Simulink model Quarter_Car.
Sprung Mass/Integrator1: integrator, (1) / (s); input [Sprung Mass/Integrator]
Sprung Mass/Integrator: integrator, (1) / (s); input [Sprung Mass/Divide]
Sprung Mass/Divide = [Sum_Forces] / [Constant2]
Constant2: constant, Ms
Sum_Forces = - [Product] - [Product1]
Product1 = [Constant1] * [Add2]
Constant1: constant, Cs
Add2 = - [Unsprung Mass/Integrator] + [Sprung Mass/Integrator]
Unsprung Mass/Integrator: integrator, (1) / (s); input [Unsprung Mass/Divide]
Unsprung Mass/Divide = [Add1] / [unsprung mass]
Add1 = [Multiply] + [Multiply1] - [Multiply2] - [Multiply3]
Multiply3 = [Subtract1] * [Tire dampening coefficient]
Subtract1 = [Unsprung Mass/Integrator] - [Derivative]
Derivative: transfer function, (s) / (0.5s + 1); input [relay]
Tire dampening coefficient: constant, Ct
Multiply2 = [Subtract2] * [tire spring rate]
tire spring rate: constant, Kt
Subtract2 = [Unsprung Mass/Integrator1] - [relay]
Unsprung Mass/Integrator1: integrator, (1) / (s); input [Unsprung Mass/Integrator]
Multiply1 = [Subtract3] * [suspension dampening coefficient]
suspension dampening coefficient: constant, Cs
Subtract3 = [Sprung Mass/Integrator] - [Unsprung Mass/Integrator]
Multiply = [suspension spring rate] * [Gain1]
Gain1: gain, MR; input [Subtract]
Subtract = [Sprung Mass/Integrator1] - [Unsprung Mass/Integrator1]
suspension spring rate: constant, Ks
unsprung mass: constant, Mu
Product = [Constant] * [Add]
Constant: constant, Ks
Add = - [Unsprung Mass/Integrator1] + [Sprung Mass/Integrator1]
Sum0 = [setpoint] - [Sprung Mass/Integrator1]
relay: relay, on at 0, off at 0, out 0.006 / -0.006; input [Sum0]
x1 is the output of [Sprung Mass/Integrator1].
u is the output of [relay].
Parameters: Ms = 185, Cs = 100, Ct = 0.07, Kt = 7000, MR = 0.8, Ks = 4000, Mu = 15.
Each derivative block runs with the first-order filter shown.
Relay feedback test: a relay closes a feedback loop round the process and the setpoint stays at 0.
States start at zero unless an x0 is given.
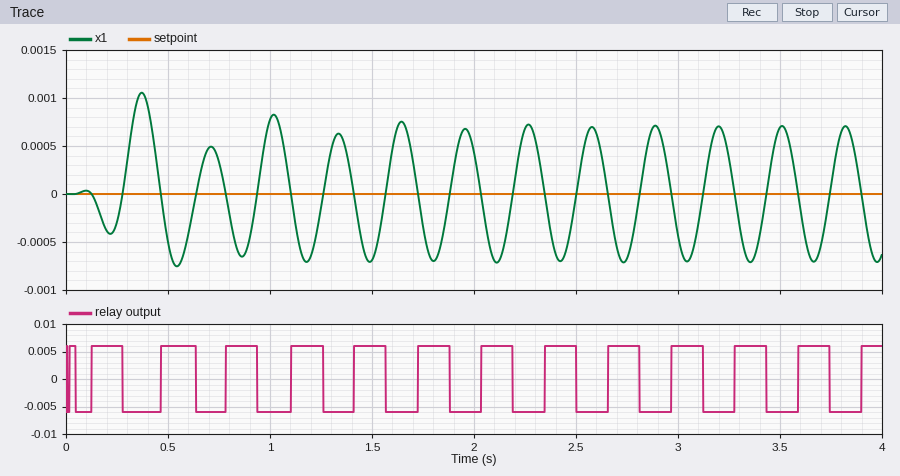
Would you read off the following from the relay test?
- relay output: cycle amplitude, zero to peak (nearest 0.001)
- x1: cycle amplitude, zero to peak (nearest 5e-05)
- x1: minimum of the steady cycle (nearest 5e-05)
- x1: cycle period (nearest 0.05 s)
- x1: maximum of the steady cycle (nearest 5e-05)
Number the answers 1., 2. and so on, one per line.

1. 0.006
2. 0.00070
3. -0.00070
4. 0.30 s
5. 0.00070
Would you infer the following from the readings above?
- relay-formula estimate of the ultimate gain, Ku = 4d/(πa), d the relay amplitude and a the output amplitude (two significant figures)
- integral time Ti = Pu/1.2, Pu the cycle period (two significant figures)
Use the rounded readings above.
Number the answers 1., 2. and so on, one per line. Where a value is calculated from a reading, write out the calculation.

1. 4 × 0.006 / (π × 0.0007) = 11
2. 0.3 / 1.2 = 0.25 s
